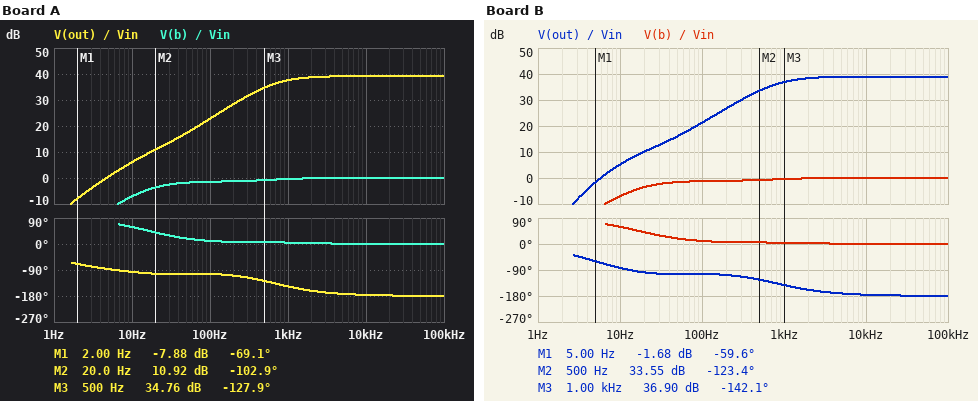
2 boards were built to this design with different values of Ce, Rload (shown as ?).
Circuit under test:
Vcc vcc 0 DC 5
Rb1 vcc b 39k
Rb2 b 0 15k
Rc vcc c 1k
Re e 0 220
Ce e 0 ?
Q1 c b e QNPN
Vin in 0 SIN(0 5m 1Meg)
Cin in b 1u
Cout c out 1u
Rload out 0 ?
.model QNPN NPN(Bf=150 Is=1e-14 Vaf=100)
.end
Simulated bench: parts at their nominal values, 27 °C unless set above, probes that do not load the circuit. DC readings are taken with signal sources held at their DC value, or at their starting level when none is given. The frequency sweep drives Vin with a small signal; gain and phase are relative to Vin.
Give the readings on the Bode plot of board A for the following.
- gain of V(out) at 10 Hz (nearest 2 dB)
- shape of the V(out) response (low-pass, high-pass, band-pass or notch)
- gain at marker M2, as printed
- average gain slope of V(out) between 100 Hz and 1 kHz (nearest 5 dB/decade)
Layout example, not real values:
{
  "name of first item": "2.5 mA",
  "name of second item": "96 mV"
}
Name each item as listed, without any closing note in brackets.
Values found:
{
  "gain of V(out) at 10 Hz": "6 dB",
  "shape of the V(out) response": "high-pass",
  "gain at marker M2, as printed": "10.92 dB",
  "average gain slope of V(out) between 100 Hz and 1 kHz": "15 dB/decade"
}
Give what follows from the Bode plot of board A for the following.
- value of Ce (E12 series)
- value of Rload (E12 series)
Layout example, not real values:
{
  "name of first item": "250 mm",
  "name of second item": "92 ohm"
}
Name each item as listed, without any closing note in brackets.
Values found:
{
  "value of Ce": "27 µF",
  "value of Rload": "180 kΩ"
}
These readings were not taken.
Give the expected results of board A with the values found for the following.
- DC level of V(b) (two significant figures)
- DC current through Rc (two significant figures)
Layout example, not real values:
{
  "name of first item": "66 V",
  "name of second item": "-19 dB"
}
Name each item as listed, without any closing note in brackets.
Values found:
{
  "DC level of V(b)": "1.2 V",
  "DC current through Rc": "2.4 mA"
}
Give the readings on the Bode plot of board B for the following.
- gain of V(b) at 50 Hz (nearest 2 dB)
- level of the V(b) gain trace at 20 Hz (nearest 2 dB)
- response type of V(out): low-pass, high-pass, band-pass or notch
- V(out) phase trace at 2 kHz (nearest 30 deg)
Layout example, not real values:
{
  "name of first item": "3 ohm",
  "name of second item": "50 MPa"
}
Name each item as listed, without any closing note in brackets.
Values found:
{
  "gain of V(b) at 50 Hz": "-2 dB",
  "level of the V(b) gain trace at 20 Hz": "-4 dB",
  "response type of V(out): low-pass, high-pass, band-pass or notch": "high-pass",
  "V(out) phase trace at 2 kHz": "-150 deg"
}
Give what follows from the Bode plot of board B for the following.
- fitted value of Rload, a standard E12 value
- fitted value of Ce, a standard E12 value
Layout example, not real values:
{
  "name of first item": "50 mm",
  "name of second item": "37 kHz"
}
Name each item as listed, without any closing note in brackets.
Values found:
{
  "fitted value of Rload, a standard E12 value": "39 kΩ",
  "fitted value of Ce, a standard E12 value": "22 µF"
}
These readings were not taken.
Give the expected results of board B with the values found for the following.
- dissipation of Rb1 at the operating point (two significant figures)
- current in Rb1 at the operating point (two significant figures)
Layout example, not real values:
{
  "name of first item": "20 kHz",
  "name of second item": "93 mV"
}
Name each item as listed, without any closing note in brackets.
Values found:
{
  "dissipation of Rb1 at the operating point": "370 µW",
  "current in Rb1 at the operating point": "97 µA"
}
